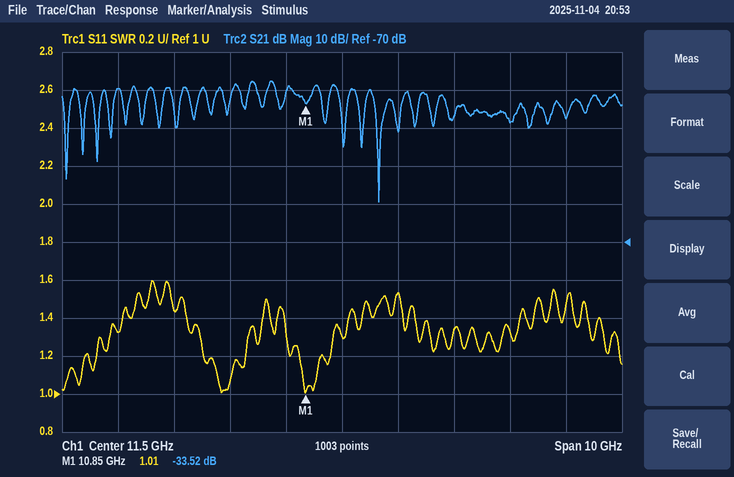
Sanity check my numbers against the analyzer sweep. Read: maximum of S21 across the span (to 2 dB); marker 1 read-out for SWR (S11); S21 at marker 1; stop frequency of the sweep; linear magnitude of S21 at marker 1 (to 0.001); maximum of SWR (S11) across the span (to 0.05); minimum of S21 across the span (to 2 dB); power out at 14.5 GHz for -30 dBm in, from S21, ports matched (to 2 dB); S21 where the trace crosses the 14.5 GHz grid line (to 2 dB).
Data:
-28 dB
1.01
-33.52 dB
16.5 GHz
0.021
1.60
-60 dB
-68 dBm
-38 dB
